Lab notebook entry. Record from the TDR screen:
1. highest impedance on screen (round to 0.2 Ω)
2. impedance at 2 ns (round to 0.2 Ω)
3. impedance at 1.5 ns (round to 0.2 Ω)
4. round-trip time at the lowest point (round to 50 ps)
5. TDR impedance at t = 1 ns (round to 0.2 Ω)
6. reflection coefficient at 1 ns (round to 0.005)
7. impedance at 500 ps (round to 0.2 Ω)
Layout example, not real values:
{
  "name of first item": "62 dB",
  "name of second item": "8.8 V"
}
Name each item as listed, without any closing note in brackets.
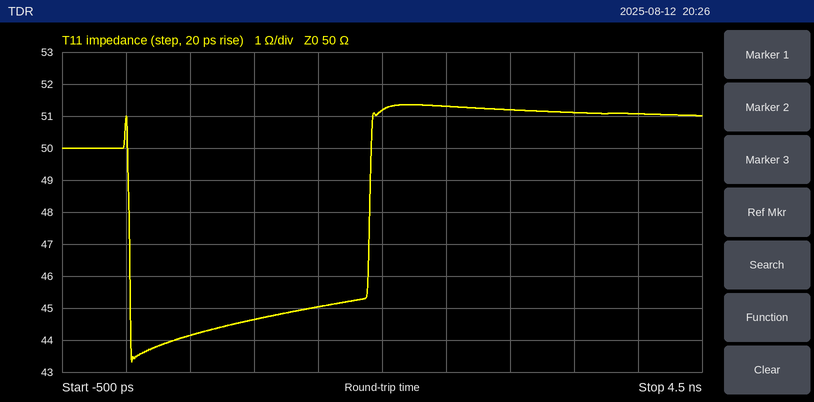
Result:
{
  "highest impedance on screen": "51.4 Ω",
  "impedance at 2 ns": "51.2 Ω",
  "impedance at 1.5 ns": "45.0 Ω",
  "round-trip time at the lowest point": "50 ps",
  "TDR impedance at t = 1 ns": "44.6 Ω",
  "reflection coefficient at 1 ns": "-0.055",
  "impedance at 500 ps": "44.2 Ω"
}
